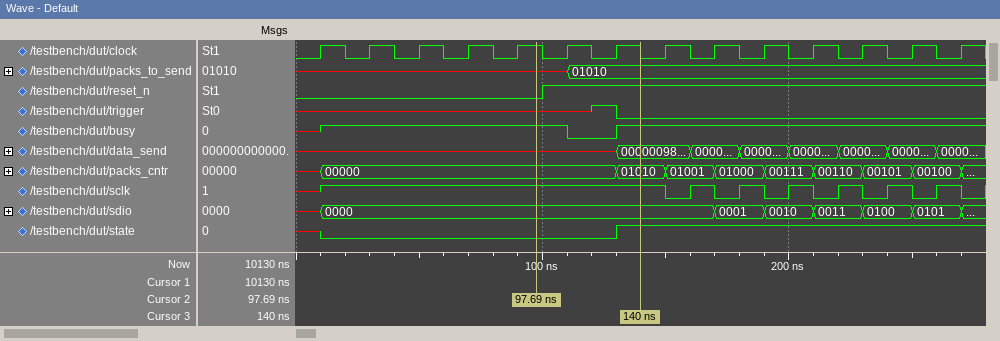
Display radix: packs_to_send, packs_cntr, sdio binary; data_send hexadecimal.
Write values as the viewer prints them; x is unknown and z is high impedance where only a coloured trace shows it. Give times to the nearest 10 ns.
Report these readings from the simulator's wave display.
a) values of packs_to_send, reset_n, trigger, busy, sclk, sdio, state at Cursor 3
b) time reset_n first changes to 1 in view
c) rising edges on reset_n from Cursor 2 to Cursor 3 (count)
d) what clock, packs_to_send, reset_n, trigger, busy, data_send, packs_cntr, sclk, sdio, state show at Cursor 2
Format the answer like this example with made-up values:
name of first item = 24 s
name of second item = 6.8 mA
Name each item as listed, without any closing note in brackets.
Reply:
values of packs_to_send, reset_n, trigger, busy, sclk, sdio, state at Cursor 3 = packs_to_send=01010, reset_n=1, trigger=0, busy=1, sclk=1, sdio=0000, state=1
time reset_n first changes to 1 in view = 100 ns
rising edges on reset_n from Cursor 2 to Cursor 3 = 1
what clock, packs_to_send, reset_n, trigger, busy, data_send, packs_cntr, sclk, sdio, state show at Cursor 2 = clock=1, packs_to_send=x, reset_n=0, trigger=x, busy=1, data_send=x, packs_cntr=00000, sclk=1, sdio=0000, state=0
